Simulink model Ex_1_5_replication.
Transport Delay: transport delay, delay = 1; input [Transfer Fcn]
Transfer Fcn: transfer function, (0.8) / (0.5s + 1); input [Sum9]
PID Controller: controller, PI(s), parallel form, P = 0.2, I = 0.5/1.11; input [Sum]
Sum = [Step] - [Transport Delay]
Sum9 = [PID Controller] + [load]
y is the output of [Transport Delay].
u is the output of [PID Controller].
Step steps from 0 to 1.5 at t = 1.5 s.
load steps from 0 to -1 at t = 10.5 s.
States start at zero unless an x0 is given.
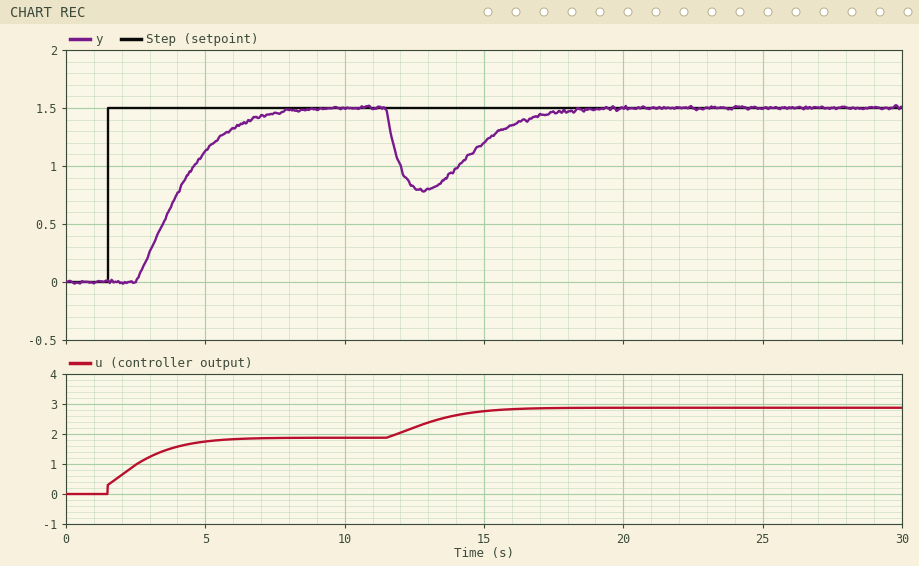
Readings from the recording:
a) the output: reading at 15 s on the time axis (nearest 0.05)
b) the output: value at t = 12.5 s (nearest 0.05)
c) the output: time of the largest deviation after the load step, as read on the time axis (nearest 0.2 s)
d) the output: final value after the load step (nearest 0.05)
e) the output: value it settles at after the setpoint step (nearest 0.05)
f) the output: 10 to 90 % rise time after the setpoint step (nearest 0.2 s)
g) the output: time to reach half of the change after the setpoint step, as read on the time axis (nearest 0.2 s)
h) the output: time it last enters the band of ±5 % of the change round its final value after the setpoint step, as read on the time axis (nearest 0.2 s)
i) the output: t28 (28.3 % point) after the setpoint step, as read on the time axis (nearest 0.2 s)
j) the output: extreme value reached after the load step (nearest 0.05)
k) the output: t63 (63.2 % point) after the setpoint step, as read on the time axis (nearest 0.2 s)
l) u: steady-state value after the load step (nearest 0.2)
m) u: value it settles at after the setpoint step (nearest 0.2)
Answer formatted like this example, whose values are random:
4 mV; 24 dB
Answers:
1.20; 0.80; 12.8 s; 1.50; 1.50; 3.4 s; 4.0 s; 7.0 s; 3.4 s; 0.80; 4.4 s; 2.8; 1.8
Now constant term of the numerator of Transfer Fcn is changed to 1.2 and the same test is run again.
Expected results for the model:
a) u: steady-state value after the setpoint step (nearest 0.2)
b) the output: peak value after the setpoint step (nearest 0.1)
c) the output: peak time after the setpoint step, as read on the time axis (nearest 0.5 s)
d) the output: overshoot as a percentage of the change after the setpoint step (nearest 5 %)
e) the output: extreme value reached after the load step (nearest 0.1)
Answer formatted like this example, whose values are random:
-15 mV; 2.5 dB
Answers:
1.2; 1.6; 6.0 s; 10 %; 0.4
